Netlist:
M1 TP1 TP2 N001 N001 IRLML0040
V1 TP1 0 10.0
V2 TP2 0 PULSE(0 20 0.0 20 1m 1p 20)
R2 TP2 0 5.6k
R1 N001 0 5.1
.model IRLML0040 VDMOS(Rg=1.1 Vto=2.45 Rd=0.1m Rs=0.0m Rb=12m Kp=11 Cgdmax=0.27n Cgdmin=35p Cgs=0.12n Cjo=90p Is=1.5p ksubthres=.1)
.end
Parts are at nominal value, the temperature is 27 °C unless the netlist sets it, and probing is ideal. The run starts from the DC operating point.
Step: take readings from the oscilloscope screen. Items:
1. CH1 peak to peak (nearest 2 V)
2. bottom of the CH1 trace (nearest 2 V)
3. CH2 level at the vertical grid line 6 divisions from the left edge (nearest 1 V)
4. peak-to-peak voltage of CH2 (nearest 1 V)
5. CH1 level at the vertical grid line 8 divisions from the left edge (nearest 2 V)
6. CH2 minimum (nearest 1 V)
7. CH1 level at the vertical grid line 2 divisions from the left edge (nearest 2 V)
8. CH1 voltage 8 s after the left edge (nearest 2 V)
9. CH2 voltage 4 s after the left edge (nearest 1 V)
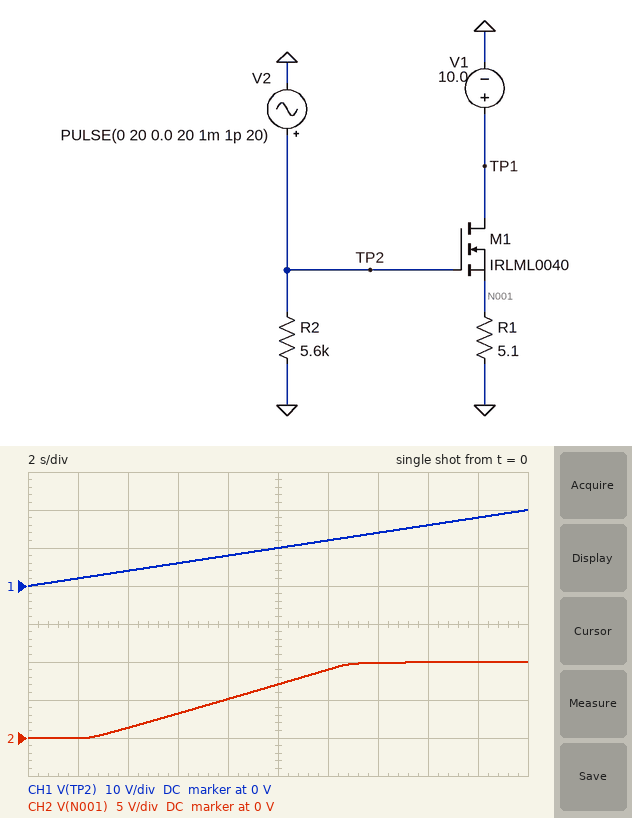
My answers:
20 V
0 V
9 V
10 V
16 V
0 V
4 V
8 V
1 V
